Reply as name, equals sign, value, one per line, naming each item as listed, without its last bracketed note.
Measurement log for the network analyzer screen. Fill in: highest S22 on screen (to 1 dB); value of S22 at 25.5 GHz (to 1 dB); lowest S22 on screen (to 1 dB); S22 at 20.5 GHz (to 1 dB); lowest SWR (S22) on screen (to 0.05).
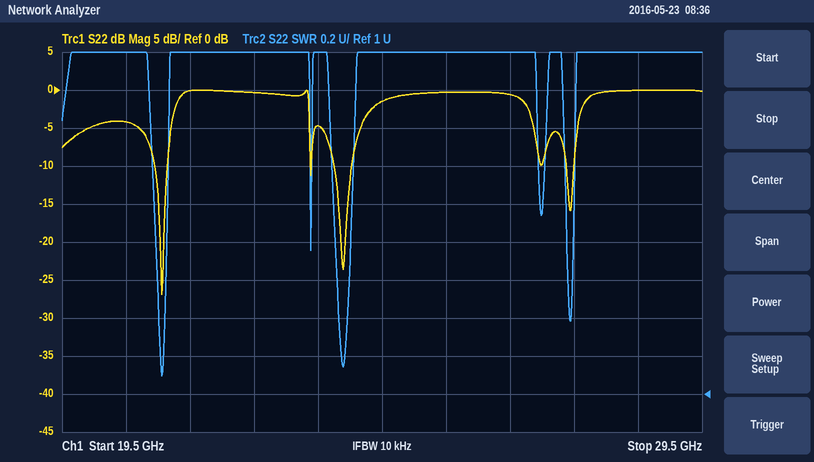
highest S22 on screen = 0 dB
value of S22 at 25.5 GHz = 0 dB
lowest S22 on screen = -27 dB
S22 at 20.5 GHz = -4 dB
lowest SWR (S22) on screen = 1.10
